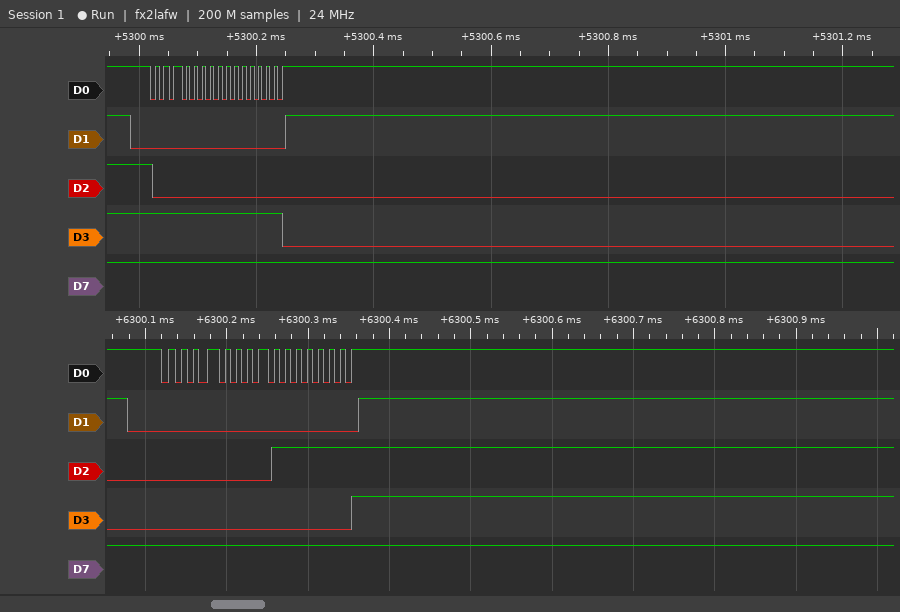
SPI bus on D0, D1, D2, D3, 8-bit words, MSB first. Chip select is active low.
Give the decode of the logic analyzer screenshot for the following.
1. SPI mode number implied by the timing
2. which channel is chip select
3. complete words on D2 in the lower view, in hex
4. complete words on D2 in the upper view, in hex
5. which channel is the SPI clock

2
D1
00, 7F
80, 00
D0
